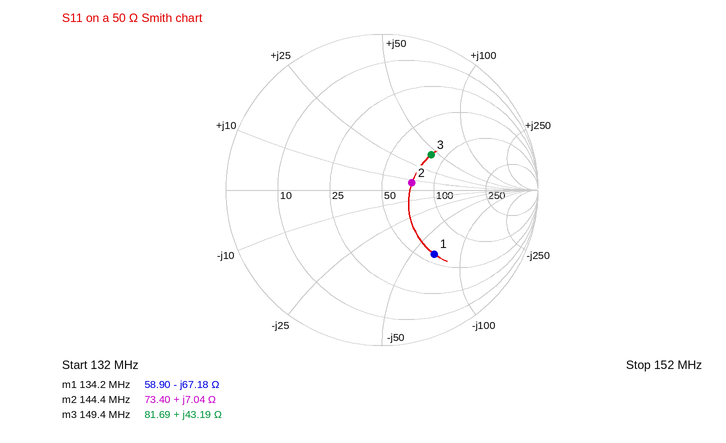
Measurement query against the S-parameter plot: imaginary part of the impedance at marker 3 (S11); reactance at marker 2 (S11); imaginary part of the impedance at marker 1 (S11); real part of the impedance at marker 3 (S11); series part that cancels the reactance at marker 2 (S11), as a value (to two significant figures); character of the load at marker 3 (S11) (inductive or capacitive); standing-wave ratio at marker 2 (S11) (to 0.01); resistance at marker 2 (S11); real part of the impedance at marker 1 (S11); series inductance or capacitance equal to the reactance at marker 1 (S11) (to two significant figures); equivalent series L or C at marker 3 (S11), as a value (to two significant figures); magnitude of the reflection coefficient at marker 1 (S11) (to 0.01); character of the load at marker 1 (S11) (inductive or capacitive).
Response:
+43.19 Ω
+7.04 Ω
-67.18 Ω
81.69 Ω
160 pF
inductive
1.49
73.40 Ω
58.90 Ω
18 pF
46 nH
0.53
capacitive
